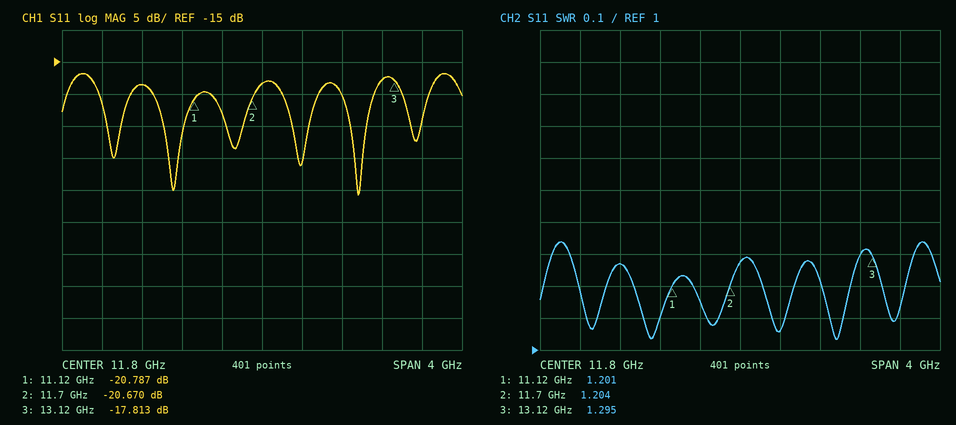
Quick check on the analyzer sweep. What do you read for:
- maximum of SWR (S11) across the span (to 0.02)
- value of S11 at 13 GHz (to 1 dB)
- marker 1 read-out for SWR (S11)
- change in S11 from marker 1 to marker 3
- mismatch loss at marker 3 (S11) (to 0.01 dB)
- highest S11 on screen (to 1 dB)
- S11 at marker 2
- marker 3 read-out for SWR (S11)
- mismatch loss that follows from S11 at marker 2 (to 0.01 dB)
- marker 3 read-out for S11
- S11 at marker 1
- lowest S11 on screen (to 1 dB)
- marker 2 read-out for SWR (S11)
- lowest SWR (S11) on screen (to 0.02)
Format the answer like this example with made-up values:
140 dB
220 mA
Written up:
1.34
-18 dB
1.201
2.974 dB
0.07 dB
-17 dB
-20.670 dB
1.295
0.04 dB
-17.813 dB
-20.787 dB
-36 dB
1.204
1.04
